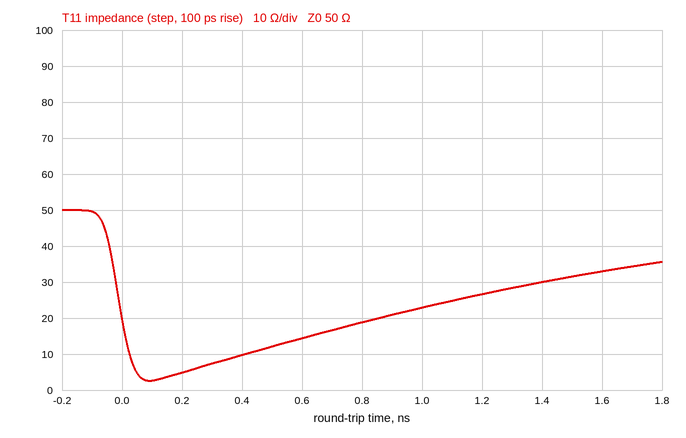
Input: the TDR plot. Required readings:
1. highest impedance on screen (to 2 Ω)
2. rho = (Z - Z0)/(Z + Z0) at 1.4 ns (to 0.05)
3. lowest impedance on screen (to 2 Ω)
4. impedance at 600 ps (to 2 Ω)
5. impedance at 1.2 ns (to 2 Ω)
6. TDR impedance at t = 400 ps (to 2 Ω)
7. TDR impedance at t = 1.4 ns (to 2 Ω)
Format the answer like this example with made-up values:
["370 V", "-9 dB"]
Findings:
["50 Ω", "-0.25", "2 Ω", "14 Ω", "26 Ω", "10 Ω", "30 Ω"]
